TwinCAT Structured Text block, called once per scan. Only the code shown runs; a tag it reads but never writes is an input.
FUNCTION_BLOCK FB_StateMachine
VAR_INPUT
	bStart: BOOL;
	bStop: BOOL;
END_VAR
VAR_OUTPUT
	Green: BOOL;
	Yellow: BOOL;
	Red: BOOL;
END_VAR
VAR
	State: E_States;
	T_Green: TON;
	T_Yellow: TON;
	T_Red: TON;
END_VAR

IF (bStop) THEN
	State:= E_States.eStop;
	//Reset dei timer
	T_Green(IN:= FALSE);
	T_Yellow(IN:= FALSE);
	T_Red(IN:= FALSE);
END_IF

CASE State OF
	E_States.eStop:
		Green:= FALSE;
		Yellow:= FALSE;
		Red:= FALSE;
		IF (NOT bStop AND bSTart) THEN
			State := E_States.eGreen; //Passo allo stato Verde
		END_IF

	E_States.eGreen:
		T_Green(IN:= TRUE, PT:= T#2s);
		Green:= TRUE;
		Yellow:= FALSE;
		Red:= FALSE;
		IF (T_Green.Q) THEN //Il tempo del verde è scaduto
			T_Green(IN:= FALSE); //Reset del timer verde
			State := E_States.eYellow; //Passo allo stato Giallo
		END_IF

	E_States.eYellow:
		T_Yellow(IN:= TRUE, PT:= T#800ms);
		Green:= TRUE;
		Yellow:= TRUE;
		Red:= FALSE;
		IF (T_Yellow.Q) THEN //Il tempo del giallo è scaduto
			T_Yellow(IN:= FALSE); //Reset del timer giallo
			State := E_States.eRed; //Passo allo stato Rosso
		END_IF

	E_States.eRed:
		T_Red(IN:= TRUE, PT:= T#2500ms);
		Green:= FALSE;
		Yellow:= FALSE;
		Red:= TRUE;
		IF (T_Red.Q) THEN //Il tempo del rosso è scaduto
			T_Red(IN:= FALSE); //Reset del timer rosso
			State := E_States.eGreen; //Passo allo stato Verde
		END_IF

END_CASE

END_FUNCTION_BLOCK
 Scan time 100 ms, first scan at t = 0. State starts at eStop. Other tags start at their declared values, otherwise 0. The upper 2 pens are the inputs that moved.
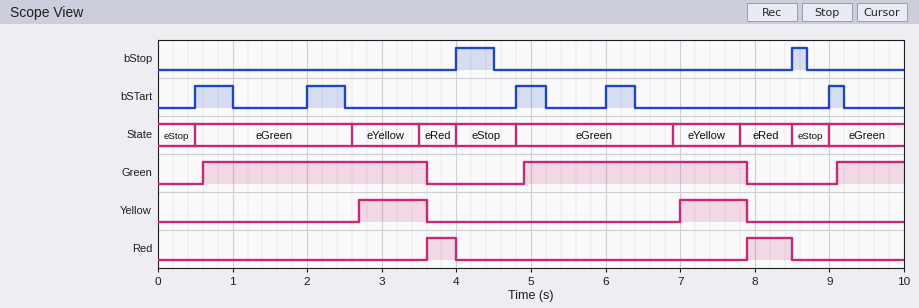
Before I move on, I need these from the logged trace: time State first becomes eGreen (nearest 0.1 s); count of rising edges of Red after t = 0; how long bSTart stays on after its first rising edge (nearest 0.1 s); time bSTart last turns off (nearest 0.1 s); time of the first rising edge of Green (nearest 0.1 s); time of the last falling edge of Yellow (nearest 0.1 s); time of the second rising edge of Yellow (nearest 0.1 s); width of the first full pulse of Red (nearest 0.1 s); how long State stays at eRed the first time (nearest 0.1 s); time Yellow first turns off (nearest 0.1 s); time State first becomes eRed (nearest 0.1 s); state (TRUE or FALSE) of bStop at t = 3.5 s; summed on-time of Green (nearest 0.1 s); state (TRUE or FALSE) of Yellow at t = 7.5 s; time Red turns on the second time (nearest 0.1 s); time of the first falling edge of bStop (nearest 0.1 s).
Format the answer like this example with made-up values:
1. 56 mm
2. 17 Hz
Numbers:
1. 0.5 s
2. 2
3. 0.5 s
4. 9.2 s
5. 0.6 s
6. 7.9 s
7. 7.0 s
8. 0.4 s
9. 0.5 s
10. 3.6 s
11. 3.5 s
12. FALSE
13. 6.9 s
14. TRUE
15. 7.9 s
16. 4.5 s
